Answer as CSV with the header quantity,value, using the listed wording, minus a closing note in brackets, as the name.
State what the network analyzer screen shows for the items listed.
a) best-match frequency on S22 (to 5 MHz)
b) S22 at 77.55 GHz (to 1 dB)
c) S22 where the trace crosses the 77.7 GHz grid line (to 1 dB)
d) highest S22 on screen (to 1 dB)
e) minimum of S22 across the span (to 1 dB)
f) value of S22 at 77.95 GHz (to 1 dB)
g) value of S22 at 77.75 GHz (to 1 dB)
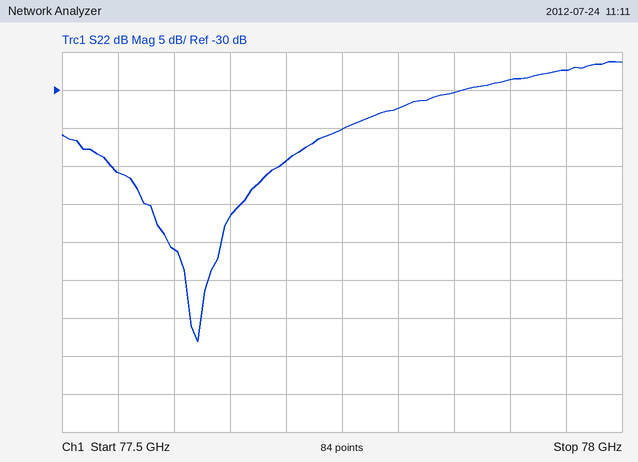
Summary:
quantity,value
best-match frequency on S22,77.620 GHz
S22 at 77.55 GHz,-41 dB
S22 where the trace crosses the 77.7 GHz grid line,-39 dB
highest S22 on screen,-26 dB
minimum of S22 across the span,-63 dB
value of S22 at 77.95 GHz,-27 dB
value of S22 at 77.75 GHz,-35 dB
